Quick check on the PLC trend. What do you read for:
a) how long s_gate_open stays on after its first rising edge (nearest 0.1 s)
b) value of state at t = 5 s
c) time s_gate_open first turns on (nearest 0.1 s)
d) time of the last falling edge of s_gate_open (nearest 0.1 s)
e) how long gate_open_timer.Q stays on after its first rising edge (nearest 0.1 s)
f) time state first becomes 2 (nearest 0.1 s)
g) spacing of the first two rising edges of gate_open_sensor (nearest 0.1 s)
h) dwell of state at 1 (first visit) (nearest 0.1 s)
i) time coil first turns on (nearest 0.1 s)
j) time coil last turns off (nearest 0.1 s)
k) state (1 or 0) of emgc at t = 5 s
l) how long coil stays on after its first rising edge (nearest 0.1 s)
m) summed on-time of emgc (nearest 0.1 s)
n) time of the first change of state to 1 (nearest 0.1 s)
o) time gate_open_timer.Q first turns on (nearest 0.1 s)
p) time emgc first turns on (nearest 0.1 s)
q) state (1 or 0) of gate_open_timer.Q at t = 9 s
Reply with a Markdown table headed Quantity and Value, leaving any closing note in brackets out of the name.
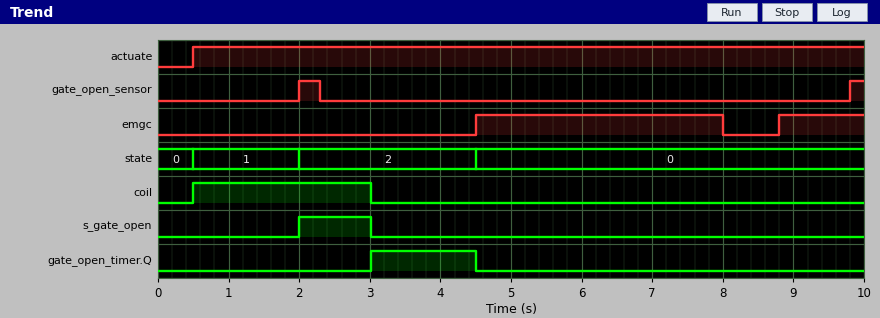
| Quantity | Value |
|---|---|
| how long s_gate_open stays on after its first rising edge | 1.0 s |
| value of state at t = 5 s | 0 |
| time s_gate_open first turns on | 2.0 s |
| time of the last falling edge of s_gate_open | 3.0 s |
| how long gate_open_timer.Q stays on after its first rising edge | 1.5 s |
| time state first becomes 2 | 2.0 s |
| spacing of the first two rising edges of gate_open_sensor | 7.8 s |
| dwell of state at 1 (first visit) | 1.5 s |
| time coil first turns on | 0.5 s |
| time coil last turns off | 3.0 s |
| state (1 or 0) of emgc at t = 5 s | 1 |
| how long coil stays on after its first rising edge | 2.5 s |
| summed on-time of emgc | 4.7 s |
| time of the first change of state to 1 | 0.5 s |
| time gate_open_timer.Q first turns on | 3.0 s |
| time emgc first turns on | 4.5 s |
| state (1 or 0) of gate_open_timer.Q at t = 9 s | 0 |
